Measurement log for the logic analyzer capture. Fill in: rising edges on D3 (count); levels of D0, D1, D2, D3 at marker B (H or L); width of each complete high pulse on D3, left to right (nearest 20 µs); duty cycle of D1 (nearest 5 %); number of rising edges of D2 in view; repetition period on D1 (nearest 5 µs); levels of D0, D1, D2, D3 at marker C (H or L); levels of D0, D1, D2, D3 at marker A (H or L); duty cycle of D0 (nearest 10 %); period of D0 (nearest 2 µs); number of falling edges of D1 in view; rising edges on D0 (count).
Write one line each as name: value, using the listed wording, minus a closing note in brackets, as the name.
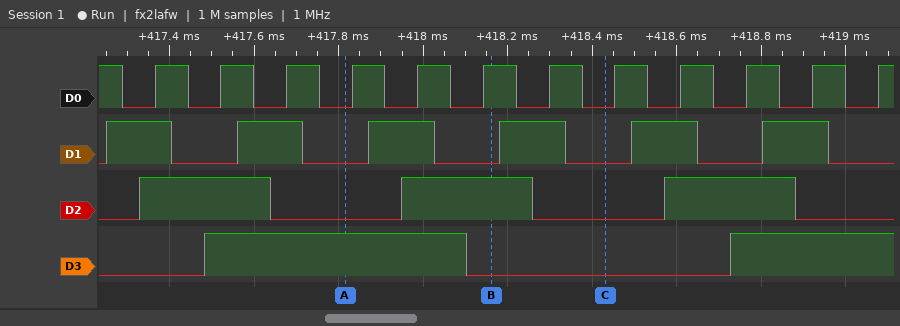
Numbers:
rising edges on D3: 2
levels of D0, D1, D2, D3 at marker B: D0=H, D1=L, D2=H, D3=L
width of each complete high pulse on D3, left to right: 620 µs
duty cycle of D1: 50 %
number of rising edges of D2 in view: 3
repetition period on D1: 310 µs
levels of D0, D1, D2, D3 at marker C: D0=L, D1=L, D2=L, D3=L
levels of D0, D1, D2, D3 at marker A: D0=L, D1=L, D2=L, D3=H
duty cycle of D0: 50 %
period of D0: 156 µs
number of falling edges of D1 in view: 6
rising edges on D0: 12
